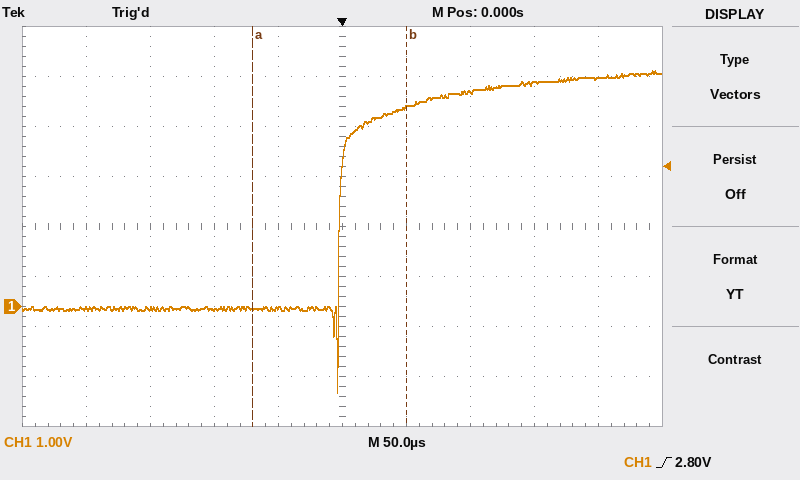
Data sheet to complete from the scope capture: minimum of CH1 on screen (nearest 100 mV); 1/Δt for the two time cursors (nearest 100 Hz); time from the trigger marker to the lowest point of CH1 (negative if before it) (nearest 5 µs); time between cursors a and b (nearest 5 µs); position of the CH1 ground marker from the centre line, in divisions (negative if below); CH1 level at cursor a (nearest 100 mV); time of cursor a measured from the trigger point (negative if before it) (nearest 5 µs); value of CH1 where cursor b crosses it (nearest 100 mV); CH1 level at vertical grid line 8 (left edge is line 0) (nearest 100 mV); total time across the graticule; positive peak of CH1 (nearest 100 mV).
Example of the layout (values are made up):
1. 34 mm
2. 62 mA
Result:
1. -1.7 V
2. 8.3 kHz
3. -5 µs
4. 120 µs
5. -1.6 div
6. 0.0 V
7. -70 µs
8. 4.0 V
9. 4.5 V
10. 500 µs
11. 4.7 V
